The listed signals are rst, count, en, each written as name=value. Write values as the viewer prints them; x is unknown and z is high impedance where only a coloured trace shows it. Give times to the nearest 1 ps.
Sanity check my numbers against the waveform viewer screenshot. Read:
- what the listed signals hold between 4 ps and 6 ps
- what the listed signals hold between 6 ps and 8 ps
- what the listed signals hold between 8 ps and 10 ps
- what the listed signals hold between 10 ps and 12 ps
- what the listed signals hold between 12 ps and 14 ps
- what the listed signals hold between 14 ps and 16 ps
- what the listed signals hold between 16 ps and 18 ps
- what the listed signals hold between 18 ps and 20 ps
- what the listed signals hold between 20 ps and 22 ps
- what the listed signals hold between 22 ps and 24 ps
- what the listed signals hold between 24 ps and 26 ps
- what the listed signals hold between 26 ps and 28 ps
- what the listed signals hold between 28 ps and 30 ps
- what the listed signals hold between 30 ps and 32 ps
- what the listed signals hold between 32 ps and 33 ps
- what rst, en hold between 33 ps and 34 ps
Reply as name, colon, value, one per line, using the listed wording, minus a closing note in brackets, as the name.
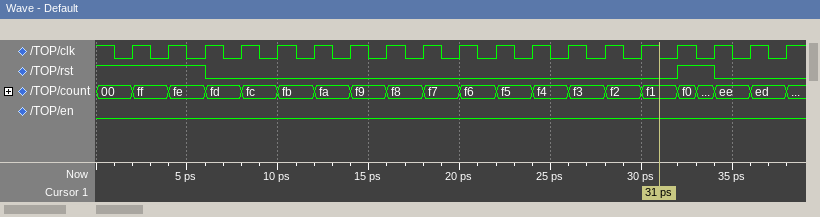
what the listed signals hold between 4 ps and 6 ps: rst=1, count=fe, en=0
what the listed signals hold between 6 ps and 8 ps: rst=0, count=fd, en=0
what the listed signals hold between 8 ps and 10 ps: rst=0, count=fc, en=0
what the listed signals hold between 10 ps and 12 ps: rst=0, count=fb, en=0
what the listed signals hold between 12 ps and 14 ps: rst=0, count=fa, en=0
what the listed signals hold between 14 ps and 16 ps: rst=0, count=f9, en=0
what the listed signals hold between 16 ps and 18 ps: rst=0, count=f8, en=0
what the listed signals hold between 18 ps and 20 ps: rst=0, count=f7, en=0
what the listed signals hold between 20 ps and 22 ps: rst=0, count=f6, en=0
what the listed signals hold between 22 ps and 24 ps: rst=0, count=f5, en=0
what the listed signals hold between 24 ps and 26 ps: rst=0, count=f4, en=0
what the listed signals hold between 26 ps and 28 ps: rst=0, count=f3, en=0
what the listed signals hold between 28 ps and 30 ps: rst=0, count=f2, en=0
what the listed signals hold between 30 ps and 32 ps: rst=0, count=f1, en=0
what the listed signals hold between 32 ps and 33 ps: rst=1, count=f0, en=0
what rst, en hold between 33 ps and 34 ps: rst=1, en=0
